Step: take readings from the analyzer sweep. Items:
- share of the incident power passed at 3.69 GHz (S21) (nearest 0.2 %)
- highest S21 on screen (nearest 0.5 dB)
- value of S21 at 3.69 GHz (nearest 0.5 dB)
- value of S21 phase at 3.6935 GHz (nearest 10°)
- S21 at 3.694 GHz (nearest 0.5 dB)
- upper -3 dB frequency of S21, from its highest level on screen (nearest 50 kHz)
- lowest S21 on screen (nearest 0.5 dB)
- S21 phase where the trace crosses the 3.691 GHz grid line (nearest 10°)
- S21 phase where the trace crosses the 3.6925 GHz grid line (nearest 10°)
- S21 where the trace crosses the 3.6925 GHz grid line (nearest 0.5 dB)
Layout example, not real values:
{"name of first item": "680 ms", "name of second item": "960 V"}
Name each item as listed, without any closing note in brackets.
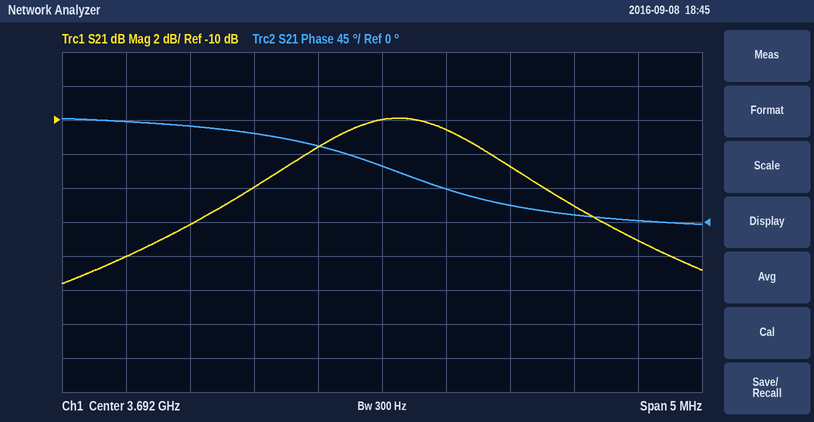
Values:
{"share of the incident power passed at 3.69 GHz (S21)": "1.6 %", "highest S21 on screen": "-10.0 dB", "value of S21 at 3.69 GHz": "-18.0 dB", "value of S21 phase at 3.6935 GHz": "10°", "S21 at 3.694 GHz": "-17.0 dB", "upper -3 dB frequency of S21, from its highest level on screen": "3.69305 GHz", "lowest S21 on screen": "-19.5 dB", "S21 phase where the trace crosses the 3.691 GHz grid line": "120°", "S21 phase where the trace crosses the 3.6925 GHz grid line": "40°", "S21 where the trace crosses the 3.6925 GHz grid line": "-10.5 dB"}
